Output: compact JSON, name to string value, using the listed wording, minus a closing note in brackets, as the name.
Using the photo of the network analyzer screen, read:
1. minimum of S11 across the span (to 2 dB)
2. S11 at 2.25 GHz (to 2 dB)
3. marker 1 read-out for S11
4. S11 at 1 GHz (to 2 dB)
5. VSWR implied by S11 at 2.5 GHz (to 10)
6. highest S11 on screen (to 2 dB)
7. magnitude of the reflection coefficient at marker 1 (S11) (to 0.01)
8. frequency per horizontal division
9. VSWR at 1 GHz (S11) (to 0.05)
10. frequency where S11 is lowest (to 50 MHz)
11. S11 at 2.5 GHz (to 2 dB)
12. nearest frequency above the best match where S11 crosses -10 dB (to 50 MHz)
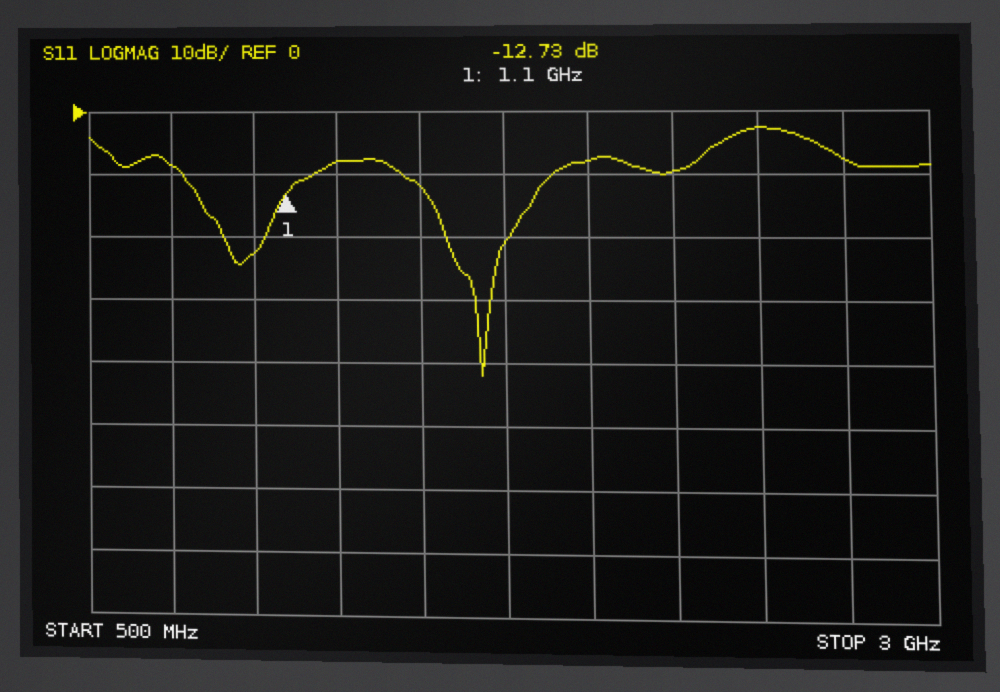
{"minimum of S11 across the span": "-42 dB", "S11 at 2.25 GHz": "-10 dB", "marker 1 read-out for S11": "-12.73 dB", "S11 at 1 GHz": "-22 dB", "VSWR implied by S11 at 2.5 GHz": "10", "highest S11 on screen": "-2 dB", "magnitude of the reflection coefficient at marker 1 (S11)": "0.23", "frequency per horizontal division": "250 MHz", "VSWR at 1 GHz (S11)": "1.15", "frequency where S11 is lowest": "1.70 GHz", "S11 at 2.5 GHz": "-2 dB", "nearest frequency above the best match where S11 crosses -10 dB": "1.90 GHz"}
